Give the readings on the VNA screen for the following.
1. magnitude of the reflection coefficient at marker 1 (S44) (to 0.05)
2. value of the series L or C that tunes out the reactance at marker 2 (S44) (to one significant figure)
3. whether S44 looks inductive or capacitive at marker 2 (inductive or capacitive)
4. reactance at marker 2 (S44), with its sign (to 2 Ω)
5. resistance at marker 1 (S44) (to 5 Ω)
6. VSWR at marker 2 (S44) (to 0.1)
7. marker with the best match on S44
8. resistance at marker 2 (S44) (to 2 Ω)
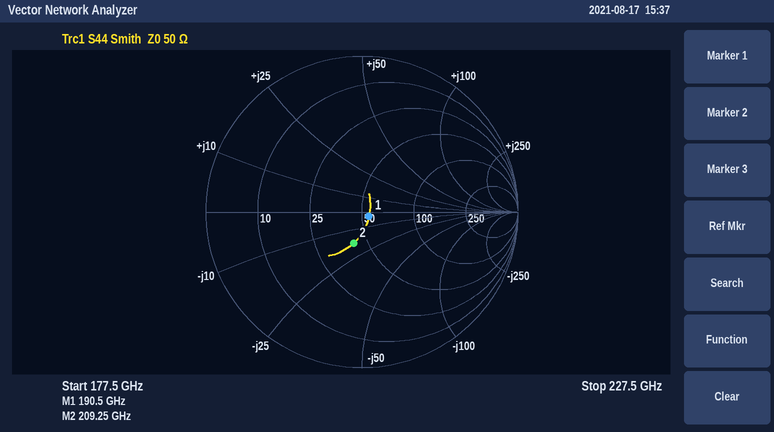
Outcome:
0.05
10 pH
capacitive
-18 Ω
55 Ω
1.5
marker 1
42 Ω
